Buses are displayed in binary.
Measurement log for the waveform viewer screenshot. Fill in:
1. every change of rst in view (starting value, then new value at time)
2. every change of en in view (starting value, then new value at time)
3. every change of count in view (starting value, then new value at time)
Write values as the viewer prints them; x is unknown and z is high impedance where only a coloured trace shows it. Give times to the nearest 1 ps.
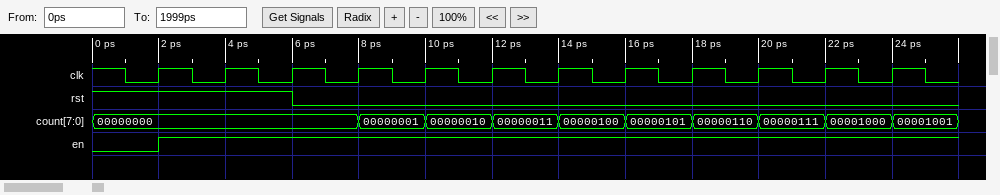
1, 0 at 6 ps
0, 1 at 2 ps
00000000, 00000001 at 8 ps, 00000010 at 10 ps, 00000011 at 12 ps, 00000100 at 14 ps, 00000101 at 16 ps, 00000110 at 18 ps, 00000111 at 20 ps, 00001000 at 22 ps, 00001001 at 24 ps
